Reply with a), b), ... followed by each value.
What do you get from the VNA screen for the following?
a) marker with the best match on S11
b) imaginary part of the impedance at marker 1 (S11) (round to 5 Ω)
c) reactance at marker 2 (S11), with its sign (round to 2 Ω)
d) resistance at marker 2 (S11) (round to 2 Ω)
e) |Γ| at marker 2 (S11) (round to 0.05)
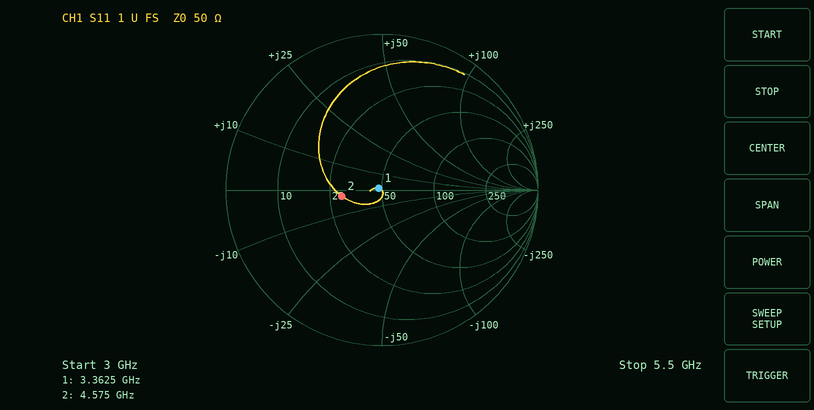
a) marker 1
b) 0 Ω
c) -2 Ω
d) 30 Ω
e) 0.25
